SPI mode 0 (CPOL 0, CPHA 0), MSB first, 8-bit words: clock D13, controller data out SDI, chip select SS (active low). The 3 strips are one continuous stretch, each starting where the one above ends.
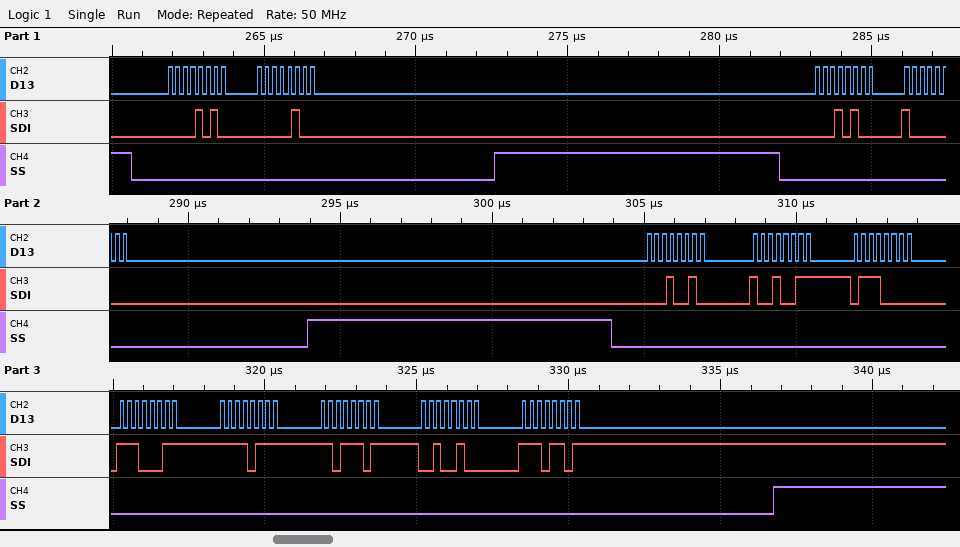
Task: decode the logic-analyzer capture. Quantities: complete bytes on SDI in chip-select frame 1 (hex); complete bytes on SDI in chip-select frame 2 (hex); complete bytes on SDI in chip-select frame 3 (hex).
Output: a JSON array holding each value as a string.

["0A 04", "14 80", "12 93 70 E3 F7 DD 24 ED"]
